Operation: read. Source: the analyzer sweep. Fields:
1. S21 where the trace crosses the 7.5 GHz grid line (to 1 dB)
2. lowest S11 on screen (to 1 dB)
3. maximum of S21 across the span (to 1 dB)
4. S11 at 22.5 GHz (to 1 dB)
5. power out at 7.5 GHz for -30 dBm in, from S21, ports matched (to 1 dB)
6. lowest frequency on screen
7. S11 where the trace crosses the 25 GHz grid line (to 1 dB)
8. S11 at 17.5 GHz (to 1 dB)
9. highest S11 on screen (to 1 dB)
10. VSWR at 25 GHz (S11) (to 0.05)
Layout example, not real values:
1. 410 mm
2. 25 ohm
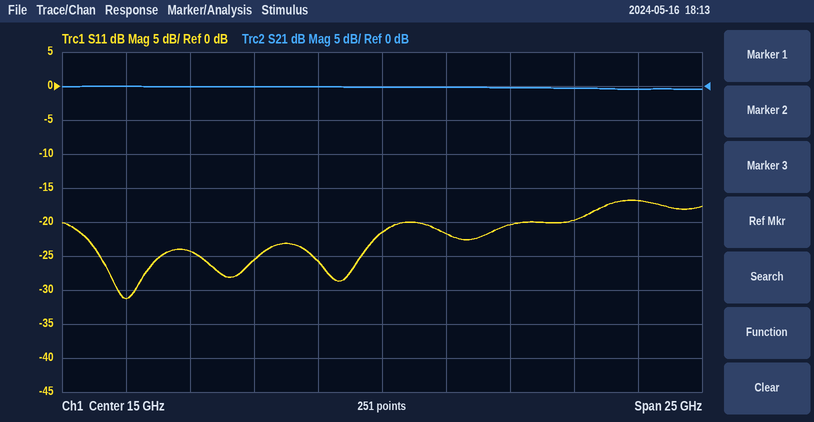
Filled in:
1. 0 dB
2. -31 dB
3. 0 dB
4. -20 dB
5. -30 dBm
6. 2.5 GHz
7. -17 dB
8. -22 dB
9. -17 dB
10. 1.35
